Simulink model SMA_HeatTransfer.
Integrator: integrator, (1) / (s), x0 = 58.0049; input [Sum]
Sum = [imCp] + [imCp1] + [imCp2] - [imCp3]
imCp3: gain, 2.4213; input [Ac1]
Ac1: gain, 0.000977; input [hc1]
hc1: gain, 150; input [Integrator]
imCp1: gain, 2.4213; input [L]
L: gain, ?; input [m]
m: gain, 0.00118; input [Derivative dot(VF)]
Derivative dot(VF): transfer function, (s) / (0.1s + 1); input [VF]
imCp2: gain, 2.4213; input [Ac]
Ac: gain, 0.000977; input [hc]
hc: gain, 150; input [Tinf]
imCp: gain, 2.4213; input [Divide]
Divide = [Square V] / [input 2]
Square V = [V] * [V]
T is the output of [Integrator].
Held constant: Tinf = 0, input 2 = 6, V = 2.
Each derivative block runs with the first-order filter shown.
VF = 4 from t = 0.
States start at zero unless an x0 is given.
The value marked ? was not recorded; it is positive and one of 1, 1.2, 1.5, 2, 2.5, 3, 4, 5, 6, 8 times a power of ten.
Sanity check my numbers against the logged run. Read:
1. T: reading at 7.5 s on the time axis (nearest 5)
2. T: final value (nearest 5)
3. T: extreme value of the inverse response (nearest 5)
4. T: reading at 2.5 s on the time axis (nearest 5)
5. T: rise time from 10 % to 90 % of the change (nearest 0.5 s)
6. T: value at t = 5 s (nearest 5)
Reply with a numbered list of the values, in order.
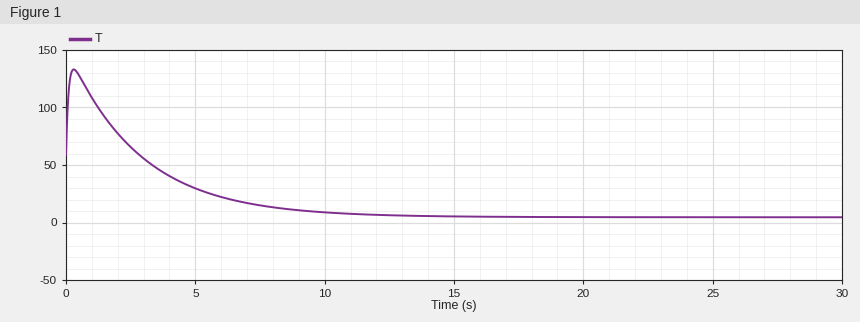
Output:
1. 15
2. 5
3. 135
4. 65
5. 6.0 s
6. 30
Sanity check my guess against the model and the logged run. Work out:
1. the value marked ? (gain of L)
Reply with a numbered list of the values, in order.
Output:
1. 8000
